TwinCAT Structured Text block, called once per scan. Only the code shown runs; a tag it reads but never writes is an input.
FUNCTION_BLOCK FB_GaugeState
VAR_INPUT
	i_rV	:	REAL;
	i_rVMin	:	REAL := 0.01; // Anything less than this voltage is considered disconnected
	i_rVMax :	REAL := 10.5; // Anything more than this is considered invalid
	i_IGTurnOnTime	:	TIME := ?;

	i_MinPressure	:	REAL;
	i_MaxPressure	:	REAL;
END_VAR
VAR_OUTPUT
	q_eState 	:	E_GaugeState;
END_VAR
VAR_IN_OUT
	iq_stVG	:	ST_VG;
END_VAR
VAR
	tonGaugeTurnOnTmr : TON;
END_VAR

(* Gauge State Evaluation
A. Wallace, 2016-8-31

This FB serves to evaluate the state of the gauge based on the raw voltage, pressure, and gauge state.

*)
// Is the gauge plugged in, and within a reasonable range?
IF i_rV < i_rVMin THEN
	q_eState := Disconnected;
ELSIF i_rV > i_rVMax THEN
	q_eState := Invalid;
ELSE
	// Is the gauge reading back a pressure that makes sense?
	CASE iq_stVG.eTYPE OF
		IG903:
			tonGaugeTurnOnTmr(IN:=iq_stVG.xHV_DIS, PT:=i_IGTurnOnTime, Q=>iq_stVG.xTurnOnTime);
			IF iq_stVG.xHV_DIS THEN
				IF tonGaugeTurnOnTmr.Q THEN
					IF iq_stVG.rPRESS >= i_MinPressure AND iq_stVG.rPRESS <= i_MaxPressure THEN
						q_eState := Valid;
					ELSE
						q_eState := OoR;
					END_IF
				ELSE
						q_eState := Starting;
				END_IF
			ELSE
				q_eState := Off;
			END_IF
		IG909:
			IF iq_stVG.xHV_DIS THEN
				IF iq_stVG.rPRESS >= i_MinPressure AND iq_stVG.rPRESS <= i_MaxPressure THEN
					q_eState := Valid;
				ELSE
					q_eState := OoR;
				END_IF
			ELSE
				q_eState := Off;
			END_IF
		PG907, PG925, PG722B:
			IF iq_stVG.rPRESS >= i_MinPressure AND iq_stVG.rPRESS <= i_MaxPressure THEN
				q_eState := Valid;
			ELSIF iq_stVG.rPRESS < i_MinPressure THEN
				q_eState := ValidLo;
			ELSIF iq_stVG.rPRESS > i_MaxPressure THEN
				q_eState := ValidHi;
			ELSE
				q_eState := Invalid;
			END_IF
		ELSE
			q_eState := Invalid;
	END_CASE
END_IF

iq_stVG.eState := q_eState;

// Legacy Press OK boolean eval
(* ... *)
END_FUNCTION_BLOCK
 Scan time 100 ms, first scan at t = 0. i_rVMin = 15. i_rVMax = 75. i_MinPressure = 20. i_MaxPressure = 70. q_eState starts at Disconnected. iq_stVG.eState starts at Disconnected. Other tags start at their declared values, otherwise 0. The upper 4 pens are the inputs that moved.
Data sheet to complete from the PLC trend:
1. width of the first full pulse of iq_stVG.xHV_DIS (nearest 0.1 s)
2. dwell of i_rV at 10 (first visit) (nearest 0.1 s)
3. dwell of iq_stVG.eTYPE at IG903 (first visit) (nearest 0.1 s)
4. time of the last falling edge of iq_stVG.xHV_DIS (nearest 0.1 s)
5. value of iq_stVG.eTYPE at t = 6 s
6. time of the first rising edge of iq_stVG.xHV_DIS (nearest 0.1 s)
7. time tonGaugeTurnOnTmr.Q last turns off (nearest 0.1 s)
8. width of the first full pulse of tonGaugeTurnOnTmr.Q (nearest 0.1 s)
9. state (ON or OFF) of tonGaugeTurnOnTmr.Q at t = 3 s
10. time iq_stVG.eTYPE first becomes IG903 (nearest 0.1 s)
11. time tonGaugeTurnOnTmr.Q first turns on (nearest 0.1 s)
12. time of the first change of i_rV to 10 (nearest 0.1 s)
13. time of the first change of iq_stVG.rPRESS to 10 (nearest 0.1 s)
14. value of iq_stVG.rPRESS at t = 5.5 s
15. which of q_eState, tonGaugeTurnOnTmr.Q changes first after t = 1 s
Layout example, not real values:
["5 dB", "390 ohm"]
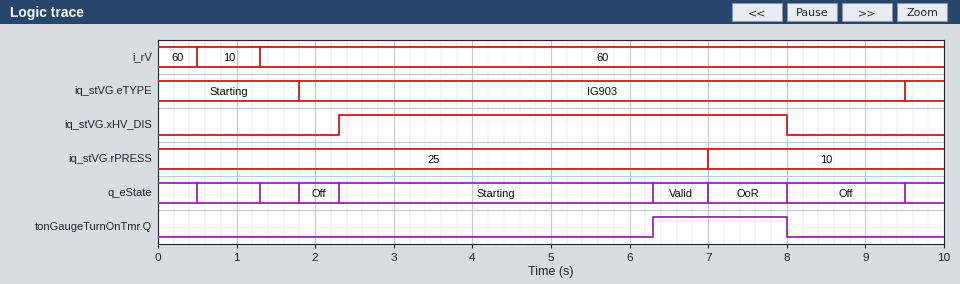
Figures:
["5.7 s", "0.8 s", "7.7 s", "8.0 s", "IG903", "2.3 s", "8.0 s", "1.7 s", "OFF", "1.8 s", "6.3 s", "0.5 s", "7.0 s", "25", "q_eState"]
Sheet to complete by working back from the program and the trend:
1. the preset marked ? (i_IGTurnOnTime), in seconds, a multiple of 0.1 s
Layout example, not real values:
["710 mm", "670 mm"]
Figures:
["4.0 s"]
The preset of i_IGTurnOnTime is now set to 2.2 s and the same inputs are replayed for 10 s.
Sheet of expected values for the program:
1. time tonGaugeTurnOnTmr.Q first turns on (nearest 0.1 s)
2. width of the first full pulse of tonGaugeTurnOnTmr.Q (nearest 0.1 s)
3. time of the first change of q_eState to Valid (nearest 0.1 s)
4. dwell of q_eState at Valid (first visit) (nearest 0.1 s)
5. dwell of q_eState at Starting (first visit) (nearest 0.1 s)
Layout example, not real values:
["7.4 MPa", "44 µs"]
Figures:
["4.5 s", "3.5 s", "4.5 s", "2.5 s", "2.2 s"]
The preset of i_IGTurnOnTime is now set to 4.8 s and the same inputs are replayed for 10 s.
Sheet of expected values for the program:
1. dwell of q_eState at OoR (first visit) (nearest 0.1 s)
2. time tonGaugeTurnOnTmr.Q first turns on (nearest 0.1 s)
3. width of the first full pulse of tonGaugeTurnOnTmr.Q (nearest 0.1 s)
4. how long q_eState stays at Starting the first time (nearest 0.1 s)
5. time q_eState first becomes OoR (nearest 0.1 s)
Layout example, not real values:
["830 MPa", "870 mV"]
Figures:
["0.9 s", "7.1 s", "0.9 s", "4.8 s", "7.1 s"]
